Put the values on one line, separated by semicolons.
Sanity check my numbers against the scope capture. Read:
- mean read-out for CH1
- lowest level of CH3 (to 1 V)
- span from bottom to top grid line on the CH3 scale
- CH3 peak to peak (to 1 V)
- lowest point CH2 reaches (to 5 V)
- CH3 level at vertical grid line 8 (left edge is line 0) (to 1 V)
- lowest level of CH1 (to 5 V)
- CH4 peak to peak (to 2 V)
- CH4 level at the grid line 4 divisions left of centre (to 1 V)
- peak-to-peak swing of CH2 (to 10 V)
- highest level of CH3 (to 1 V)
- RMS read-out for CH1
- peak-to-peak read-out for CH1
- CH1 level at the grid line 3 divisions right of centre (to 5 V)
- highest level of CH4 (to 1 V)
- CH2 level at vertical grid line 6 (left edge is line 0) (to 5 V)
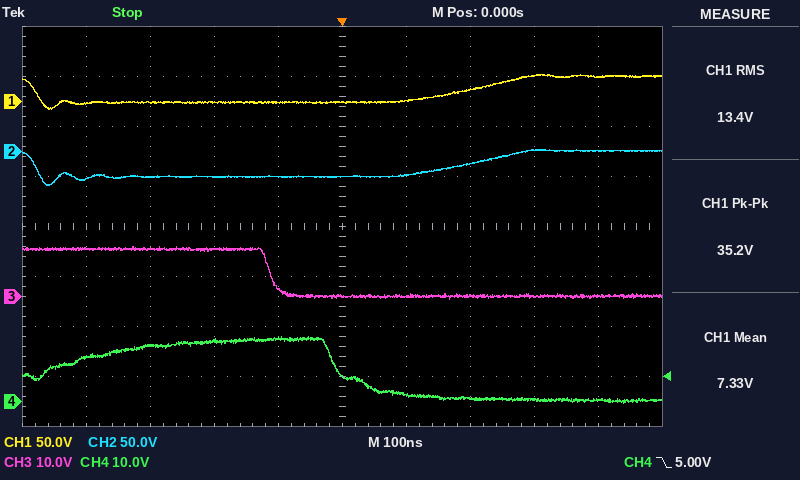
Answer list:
7.33 V; -1 V; 80 V; 11 V; -35 V; 0 V; -10 V; 14 V; 9 V; 40 V; 10 V; 13.4 V; 35.2 V; 25 V; 13 V; -25 V
